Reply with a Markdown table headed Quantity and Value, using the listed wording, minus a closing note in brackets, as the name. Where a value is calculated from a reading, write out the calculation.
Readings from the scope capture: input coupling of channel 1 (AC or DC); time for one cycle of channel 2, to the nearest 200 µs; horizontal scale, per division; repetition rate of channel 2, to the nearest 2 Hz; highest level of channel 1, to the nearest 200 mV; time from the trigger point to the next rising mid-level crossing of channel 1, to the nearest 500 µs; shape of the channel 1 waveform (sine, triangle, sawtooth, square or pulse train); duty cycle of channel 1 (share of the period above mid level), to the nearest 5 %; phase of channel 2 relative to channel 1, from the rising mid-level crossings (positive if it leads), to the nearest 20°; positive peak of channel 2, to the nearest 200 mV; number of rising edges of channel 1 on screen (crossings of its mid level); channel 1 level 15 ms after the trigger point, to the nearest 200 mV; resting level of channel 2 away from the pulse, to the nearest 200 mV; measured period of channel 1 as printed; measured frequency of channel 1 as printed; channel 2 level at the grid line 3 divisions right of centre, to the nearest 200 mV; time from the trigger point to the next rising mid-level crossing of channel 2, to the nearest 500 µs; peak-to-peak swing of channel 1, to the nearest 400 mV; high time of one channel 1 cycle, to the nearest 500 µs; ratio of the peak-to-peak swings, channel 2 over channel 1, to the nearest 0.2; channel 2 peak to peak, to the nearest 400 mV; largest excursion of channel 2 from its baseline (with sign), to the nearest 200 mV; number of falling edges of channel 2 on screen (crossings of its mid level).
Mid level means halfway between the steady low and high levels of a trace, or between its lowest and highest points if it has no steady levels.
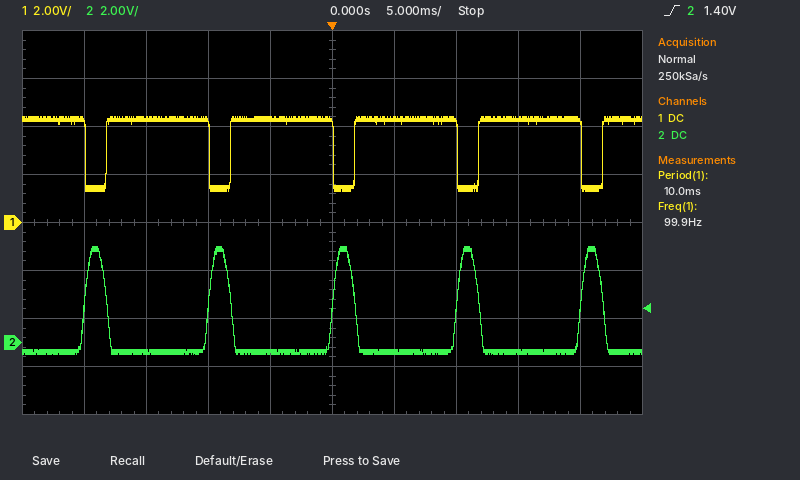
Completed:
| Quantity | Value |
|---|---|
| input coupling of channel 1 | DC |
| time for one cycle of channel 2, to the nearest 200 µs | 10.0 ms |
| horizontal scale, per division | 5 ms |
| repetition rate of channel 2, to the nearest 2 Hz | 1 / 10.0 ms ≈ 100 Hz |
| highest level of channel 1, to the nearest 200 mV | 4.4 V |
| time from the trigger point to the next rising mid-level crossing of channel 1, to the nearest 500 µs | 2.0 ms |
| shape of the channel 1 waveform | pulse train |
| duty cycle of channel 1 (share of the period above mid level), to the nearest 5 % | 85 % |
| phase of channel 2 relative to channel 1, from the rising mid-level crossings (positive if it leads), to the nearest 20° | +60° |
| positive peak of channel 2, to the nearest 200 mV | 4.0 V |
| number of rising edges of channel 1 on screen | 5 |
| channel 1 level 15 ms after the trigger point, to the nearest 200 mV | 4.4 V |
| resting level of channel 2 away from the pulse, to the nearest 200 mV | -400 mV |
| measured period of channel 1 as printed | 10.0 ms |
| measured frequency of channel 1 as printed | 99.9 Hz |
| channel 2 level at the grid line 3 divisions right of centre, to the nearest 200 mV | -400 mV |
| time from the trigger point to the next rising mid-level crossing of channel 2, to the nearest 500 µs | 10.0 ms |
| peak-to-peak swing of channel 1, to the nearest 400 mV | 3.2 V |
| high time of one channel 1 cycle, to the nearest 500 µs | 8.5 ms |
| ratio of the peak-to-peak swings, channel 2 over channel 1, to the nearest 0.2 | 4.4 V / 3.2 V ≈ 1.4 |
| channel 2 peak to peak, to the nearest 400 mV | 4.4 V |
| largest excursion of channel 2 from its baseline (with sign), to the nearest 200 mV | 4.0 V − (-400 mV) = +4.4 V |
| number of falling edges of channel 2 on screen | 5 |
